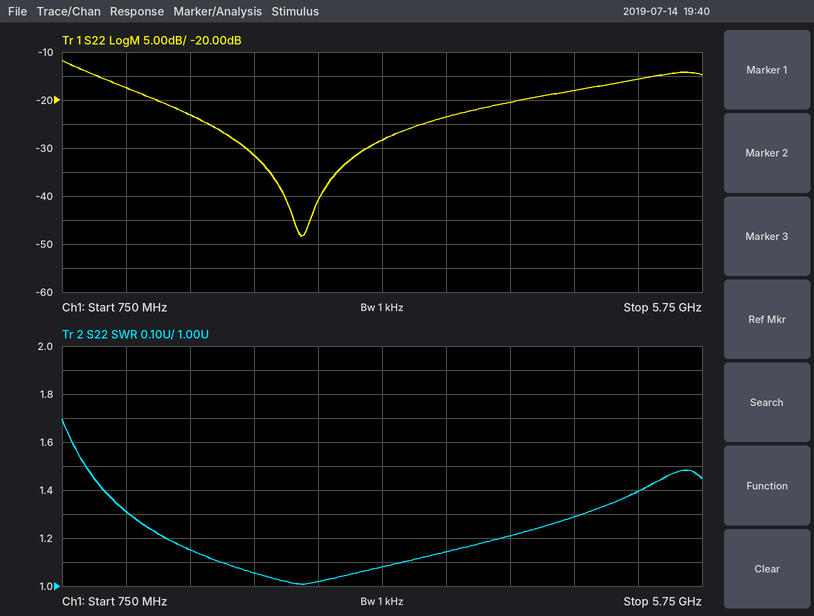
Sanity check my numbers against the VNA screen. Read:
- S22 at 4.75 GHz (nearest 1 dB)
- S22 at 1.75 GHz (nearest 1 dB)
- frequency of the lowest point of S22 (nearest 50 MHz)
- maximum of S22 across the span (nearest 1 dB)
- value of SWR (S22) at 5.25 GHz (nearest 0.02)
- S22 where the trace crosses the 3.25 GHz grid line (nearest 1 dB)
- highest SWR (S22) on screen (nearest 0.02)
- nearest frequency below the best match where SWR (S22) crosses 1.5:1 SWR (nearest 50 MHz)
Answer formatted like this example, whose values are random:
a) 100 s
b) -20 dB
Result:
a) -18 dB
b) -23 dB
c) 2.60 GHz
d) -12 dB
e) 1.40
f) -28 dB
g) 1.70
h) 950 MHz
